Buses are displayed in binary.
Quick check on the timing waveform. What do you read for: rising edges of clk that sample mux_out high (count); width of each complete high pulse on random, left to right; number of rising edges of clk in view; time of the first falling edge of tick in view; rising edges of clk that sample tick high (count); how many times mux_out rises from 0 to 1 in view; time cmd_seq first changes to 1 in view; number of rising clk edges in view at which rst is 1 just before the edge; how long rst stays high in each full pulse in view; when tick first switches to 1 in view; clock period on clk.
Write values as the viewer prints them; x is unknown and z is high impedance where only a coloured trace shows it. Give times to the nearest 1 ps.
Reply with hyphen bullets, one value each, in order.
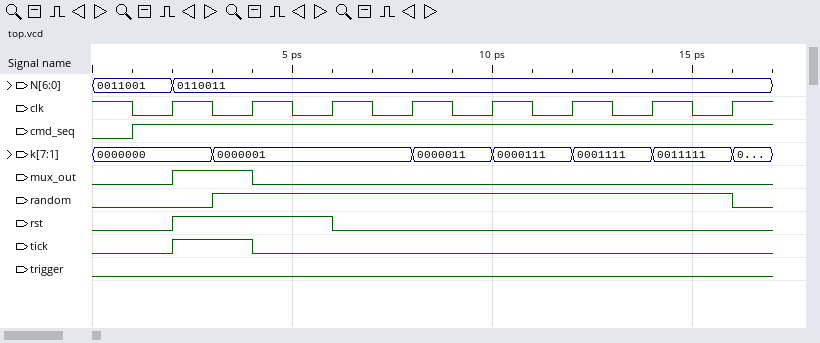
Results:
- 1
- 13 ps
- 8
- 4 ps
- 1
- 1
- 1 ps
- 2
- 4 ps
- 2 ps
- 2 ps
